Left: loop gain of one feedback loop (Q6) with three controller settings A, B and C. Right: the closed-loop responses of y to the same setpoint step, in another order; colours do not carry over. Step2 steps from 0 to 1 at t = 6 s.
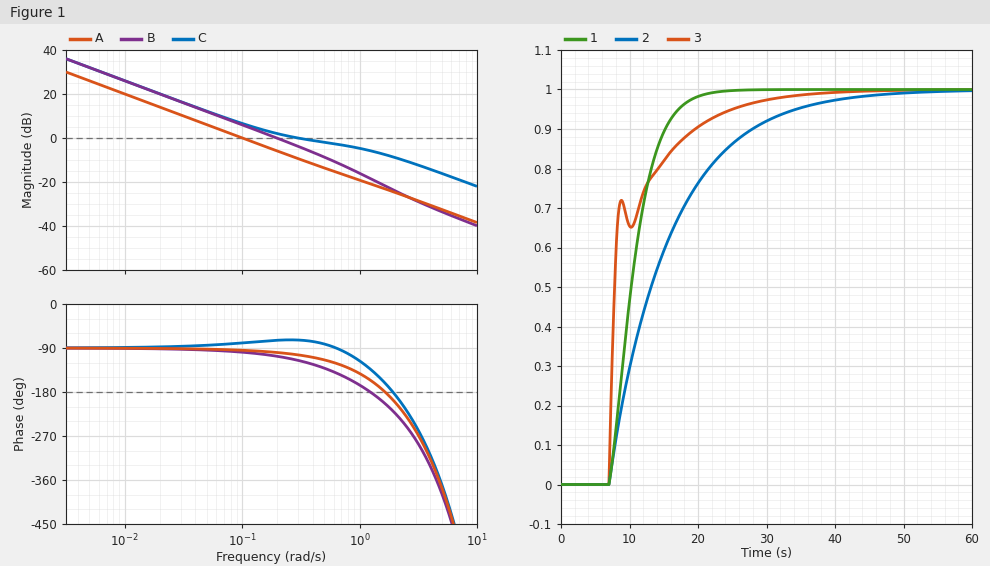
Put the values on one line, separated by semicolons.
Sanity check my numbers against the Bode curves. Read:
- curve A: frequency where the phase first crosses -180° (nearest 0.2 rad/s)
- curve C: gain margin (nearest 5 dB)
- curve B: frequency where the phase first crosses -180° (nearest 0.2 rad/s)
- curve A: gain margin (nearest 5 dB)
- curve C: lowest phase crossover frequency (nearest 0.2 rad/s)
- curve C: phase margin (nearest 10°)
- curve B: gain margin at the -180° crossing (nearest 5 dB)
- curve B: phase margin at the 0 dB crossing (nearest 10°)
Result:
1.6 rad/s; 10 dB; 1.2 rad/s; 25 dB; 2.0 rad/s; 110°; 20 dB; 70°
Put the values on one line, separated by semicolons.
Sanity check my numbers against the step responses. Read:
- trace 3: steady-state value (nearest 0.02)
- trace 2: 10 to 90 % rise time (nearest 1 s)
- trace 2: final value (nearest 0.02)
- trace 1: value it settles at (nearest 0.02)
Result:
1.00; 20 s; 1.00; 1.00
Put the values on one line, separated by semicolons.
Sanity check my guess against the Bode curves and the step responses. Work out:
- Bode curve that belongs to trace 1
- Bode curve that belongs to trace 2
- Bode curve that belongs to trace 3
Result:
B; A; C
